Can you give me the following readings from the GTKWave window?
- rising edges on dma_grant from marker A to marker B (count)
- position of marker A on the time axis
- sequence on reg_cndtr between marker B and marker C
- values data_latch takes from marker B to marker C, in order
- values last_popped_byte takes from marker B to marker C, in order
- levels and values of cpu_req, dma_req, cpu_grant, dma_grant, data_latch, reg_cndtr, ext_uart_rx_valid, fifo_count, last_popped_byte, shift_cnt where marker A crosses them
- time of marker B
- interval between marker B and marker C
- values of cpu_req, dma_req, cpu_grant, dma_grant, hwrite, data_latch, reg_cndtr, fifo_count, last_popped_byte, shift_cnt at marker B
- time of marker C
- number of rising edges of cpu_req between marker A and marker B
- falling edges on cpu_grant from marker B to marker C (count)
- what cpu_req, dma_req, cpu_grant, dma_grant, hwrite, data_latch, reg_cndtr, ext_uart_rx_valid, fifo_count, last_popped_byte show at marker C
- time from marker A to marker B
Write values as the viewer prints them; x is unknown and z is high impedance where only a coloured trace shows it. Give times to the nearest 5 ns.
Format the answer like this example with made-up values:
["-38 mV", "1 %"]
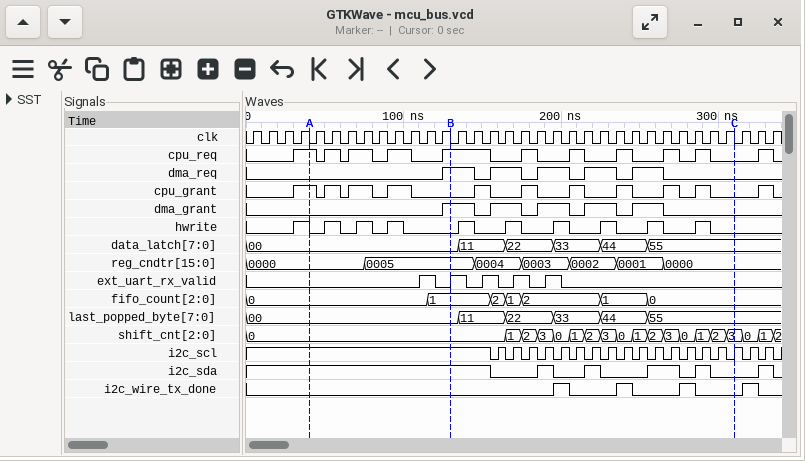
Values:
["1", "40 ns", "0005, 0004, 0003, 0002, 0001, 0000", "00, 11, 22, 33, 44, 55", "00, 11, 22, 33, 44, 55", "cpu_req=1, dma_req=0, cpu_grant=1, dma_grant=0, data_latch=00, reg_cndtr=0000, ext_uart_rx_valid=0, fifo_count=0, last_popped_byte=00, shift_cnt=0", "130 ns", "180 ns", "cpu_req=1, dma_req=1, cpu_grant=0, dma_grant=1, hwrite=0, data_latch=00, reg_cndtr=0005, fifo_count=1, last_popped_byte=00, shift_cnt=0", "310 ns", "4", "6", "cpu_req=0, dma_req=0, cpu_grant=0, dma_grant=0, hwrite=0, data_latch=55, reg_cndtr=0000, ext_uart_rx_valid=0, fifo_count=0, last_popped_byte=55", "90 ns"]
